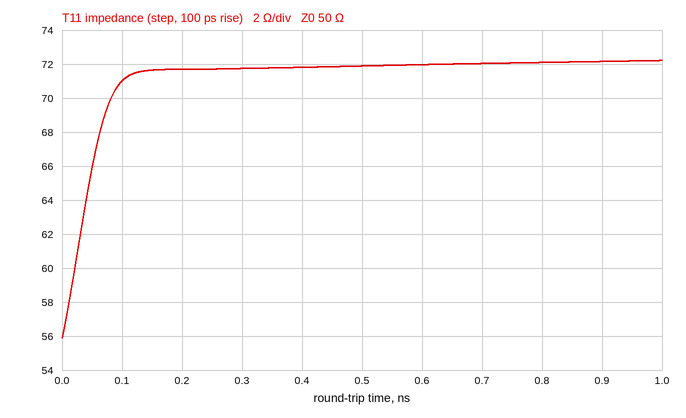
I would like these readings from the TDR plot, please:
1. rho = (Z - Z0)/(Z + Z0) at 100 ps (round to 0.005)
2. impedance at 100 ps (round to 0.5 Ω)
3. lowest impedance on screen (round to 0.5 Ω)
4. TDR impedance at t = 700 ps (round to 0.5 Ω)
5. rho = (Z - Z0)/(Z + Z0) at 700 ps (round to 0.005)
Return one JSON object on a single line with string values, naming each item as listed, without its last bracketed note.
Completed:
{"rho = (Z - Z0)/(Z + Z0) at 100 ps": "+0.175", "impedance at 100 ps": "71.0 Ω", "lowest impedance on screen": "56.0 Ω", "TDR impedance at t = 700 ps": "72.0 Ω", "rho = (Z - Z0)/(Z + Z0) at 700 ps": "+0.180"}
